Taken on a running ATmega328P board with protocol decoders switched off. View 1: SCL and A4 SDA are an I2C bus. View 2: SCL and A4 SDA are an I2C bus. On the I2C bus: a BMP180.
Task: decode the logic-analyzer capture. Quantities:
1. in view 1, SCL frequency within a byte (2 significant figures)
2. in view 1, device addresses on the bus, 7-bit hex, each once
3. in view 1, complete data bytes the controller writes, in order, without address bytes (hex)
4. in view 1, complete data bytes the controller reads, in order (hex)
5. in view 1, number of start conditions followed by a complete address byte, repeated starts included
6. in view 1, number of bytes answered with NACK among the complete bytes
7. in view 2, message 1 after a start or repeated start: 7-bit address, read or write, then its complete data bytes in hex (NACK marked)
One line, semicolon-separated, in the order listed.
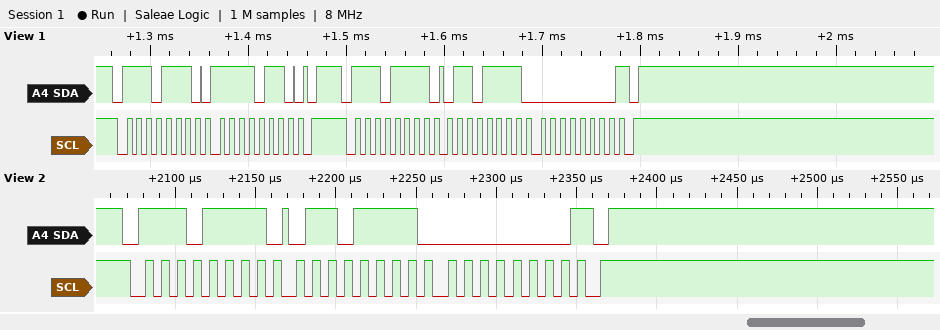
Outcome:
100 kHz; 0x77; F6; 6F 00; 2; 1; 0x77 read: 6F 00 NACK
